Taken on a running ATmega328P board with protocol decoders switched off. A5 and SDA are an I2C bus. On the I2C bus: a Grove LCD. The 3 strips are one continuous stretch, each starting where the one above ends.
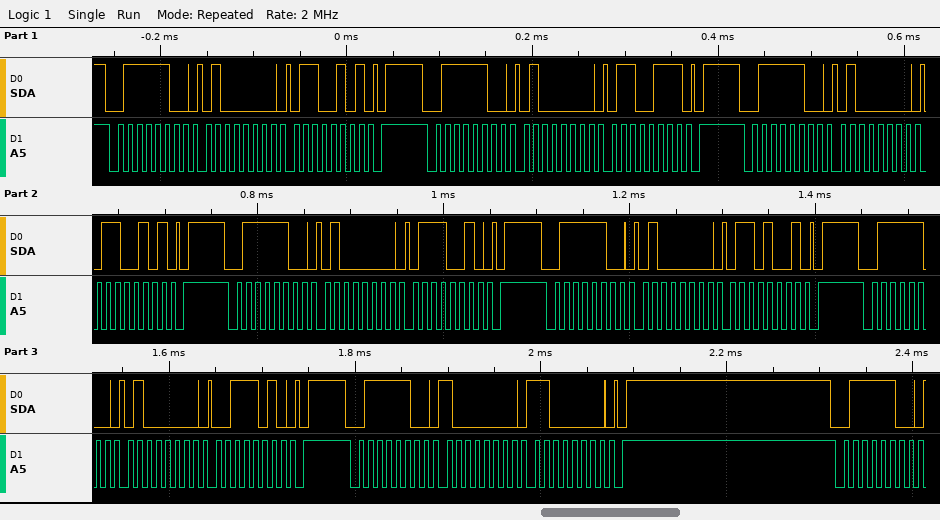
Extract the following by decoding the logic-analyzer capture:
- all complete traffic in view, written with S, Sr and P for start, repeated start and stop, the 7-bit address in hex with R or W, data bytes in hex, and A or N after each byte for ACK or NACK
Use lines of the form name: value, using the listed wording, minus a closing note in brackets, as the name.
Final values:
all complete traffic in view, written with S, Sr and P for start, repeated start and stop, the 7-bit address in hex with R or W, data bytes in hex, and A or N after each byte for ACK or NACK: S 3EW A 40 A 65 A P S 3EW A 40 A 67 A P S 3EW A 40 A 65 A P S 3EW A 40 A 72 A P S 3EW A 40 A 69 A P S 3EW A 40 A 3A A P S 3EW A 80 A C0 A P S 3EW A
